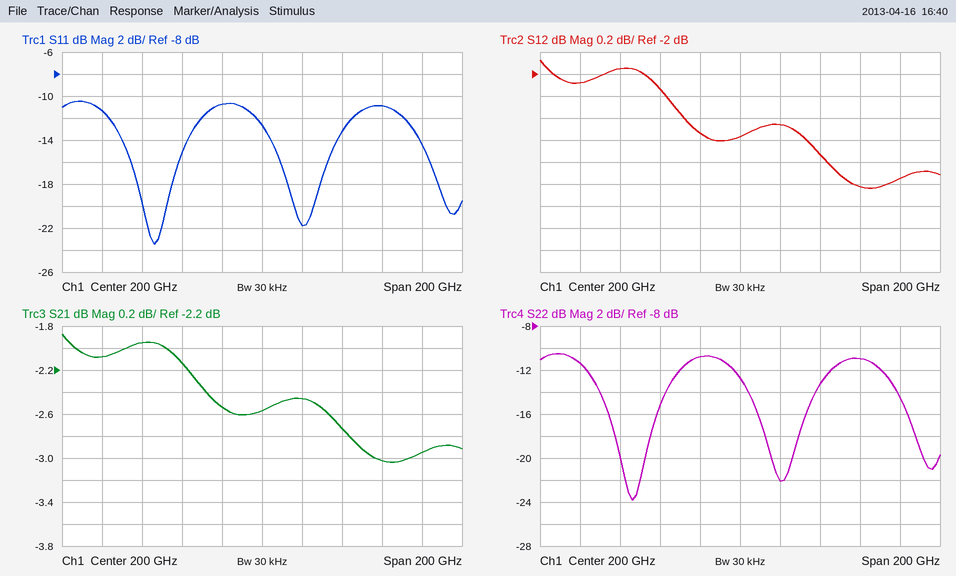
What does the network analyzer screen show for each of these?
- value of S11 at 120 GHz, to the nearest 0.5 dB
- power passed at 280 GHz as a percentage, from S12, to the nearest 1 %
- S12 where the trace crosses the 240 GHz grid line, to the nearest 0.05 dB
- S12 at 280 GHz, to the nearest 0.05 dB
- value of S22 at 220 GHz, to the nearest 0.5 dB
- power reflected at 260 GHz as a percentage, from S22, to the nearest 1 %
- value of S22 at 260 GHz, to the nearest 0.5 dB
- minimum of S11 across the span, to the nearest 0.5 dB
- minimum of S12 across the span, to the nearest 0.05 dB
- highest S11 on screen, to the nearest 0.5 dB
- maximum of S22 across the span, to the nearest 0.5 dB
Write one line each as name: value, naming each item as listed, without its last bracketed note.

value of S11 at 120 GHz, to the nearest 0.5 dB: -11.5 dB
power passed at 280 GHz as a percentage, from S12, to the nearest 1 %: 51 %
S12 where the trace crosses the 240 GHz grid line, to the nearest 0.05 dB: -2.75 dB
S12 at 280 GHz, to the nearest 0.05 dB: -2.95 dB
value of S22 at 220 GHz, to the nearest 0.5 dB: -22.0 dB
power reflected at 260 GHz as a percentage, from S22, to the nearest 1 %: 8 %
value of S22 at 260 GHz, to the nearest 0.5 dB: -11.0 dB
minimum of S11 across the span, to the nearest 0.5 dB: -23.5 dB
minimum of S12 across the span, to the nearest 0.05 dB: -3.05 dB
highest S11 on screen, to the nearest 0.5 dB: -10.5 dB
maximum of S22 across the span, to the nearest 0.5 dB: -10.5 dB
